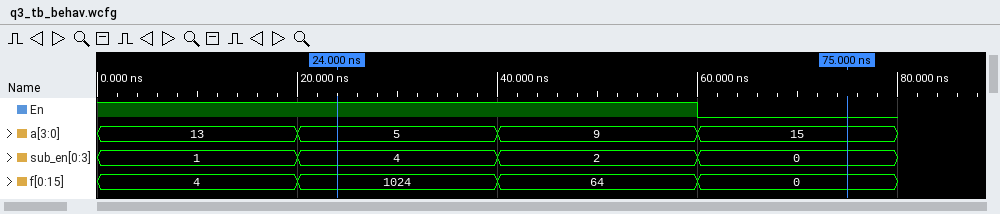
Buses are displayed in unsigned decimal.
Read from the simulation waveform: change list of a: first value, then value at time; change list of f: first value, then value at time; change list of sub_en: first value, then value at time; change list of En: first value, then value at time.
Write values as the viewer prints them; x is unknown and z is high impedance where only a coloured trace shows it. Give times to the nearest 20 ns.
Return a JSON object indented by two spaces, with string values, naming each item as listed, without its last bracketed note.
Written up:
{
  "change list of a: first value, then value at time": "13, 5 at 20 ns, 9 at 40 ns, 15 at 60 ns",
  "change list of f: first value, then value at time": "4, 1024 at 20 ns, 64 at 40 ns, 0 at 60 ns",
  "change list of sub_en: first value, then value at time": "1, 4 at 20 ns, 2 at 40 ns, 0 at 60 ns",
  "change list of En: first value, then value at time": "1, 0 at 60 ns"
}
